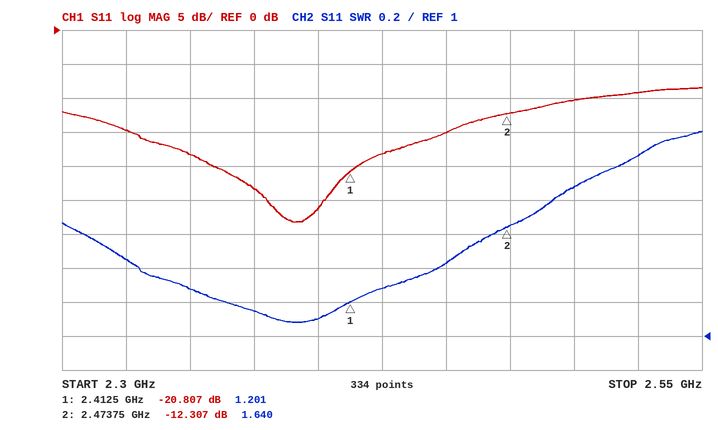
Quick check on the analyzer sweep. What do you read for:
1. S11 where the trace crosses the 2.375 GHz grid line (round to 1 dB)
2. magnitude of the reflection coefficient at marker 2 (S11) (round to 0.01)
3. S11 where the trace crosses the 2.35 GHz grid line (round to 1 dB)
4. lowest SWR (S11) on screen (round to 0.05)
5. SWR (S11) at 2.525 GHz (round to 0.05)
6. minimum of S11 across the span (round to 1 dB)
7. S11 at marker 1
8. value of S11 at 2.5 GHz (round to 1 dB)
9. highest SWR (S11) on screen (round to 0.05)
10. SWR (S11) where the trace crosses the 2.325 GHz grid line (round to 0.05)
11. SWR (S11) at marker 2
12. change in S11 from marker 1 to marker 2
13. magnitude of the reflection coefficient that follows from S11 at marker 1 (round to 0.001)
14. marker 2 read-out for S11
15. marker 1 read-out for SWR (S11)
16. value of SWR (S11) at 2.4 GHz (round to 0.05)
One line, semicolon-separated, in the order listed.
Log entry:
-23 dB; 0.24; -18 dB; 1.10; 2.05; -28 dB; -20.807 dB; -10 dB; 2.20; 1.45; 1.640; 8.500 dB; 0.091; -12.307 dB; 1.201; 1.10
